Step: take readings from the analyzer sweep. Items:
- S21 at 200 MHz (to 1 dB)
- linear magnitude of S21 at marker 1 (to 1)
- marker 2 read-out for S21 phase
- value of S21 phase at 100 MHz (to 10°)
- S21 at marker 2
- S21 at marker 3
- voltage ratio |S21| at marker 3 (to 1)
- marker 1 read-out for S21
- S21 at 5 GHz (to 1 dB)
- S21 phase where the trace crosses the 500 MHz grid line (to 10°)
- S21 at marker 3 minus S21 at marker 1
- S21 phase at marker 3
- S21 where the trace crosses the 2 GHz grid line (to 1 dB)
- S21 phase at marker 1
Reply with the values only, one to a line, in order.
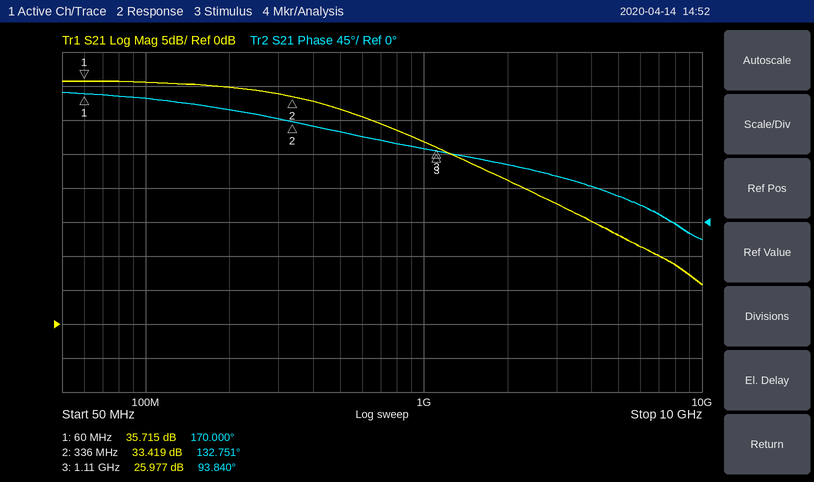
35 dB
61
132.751°
160°
33.419 dB
25.977 dB
20
35.715 dB
13 dB
120°
-9.738 dB
93.840°
21 dB
170.000°
